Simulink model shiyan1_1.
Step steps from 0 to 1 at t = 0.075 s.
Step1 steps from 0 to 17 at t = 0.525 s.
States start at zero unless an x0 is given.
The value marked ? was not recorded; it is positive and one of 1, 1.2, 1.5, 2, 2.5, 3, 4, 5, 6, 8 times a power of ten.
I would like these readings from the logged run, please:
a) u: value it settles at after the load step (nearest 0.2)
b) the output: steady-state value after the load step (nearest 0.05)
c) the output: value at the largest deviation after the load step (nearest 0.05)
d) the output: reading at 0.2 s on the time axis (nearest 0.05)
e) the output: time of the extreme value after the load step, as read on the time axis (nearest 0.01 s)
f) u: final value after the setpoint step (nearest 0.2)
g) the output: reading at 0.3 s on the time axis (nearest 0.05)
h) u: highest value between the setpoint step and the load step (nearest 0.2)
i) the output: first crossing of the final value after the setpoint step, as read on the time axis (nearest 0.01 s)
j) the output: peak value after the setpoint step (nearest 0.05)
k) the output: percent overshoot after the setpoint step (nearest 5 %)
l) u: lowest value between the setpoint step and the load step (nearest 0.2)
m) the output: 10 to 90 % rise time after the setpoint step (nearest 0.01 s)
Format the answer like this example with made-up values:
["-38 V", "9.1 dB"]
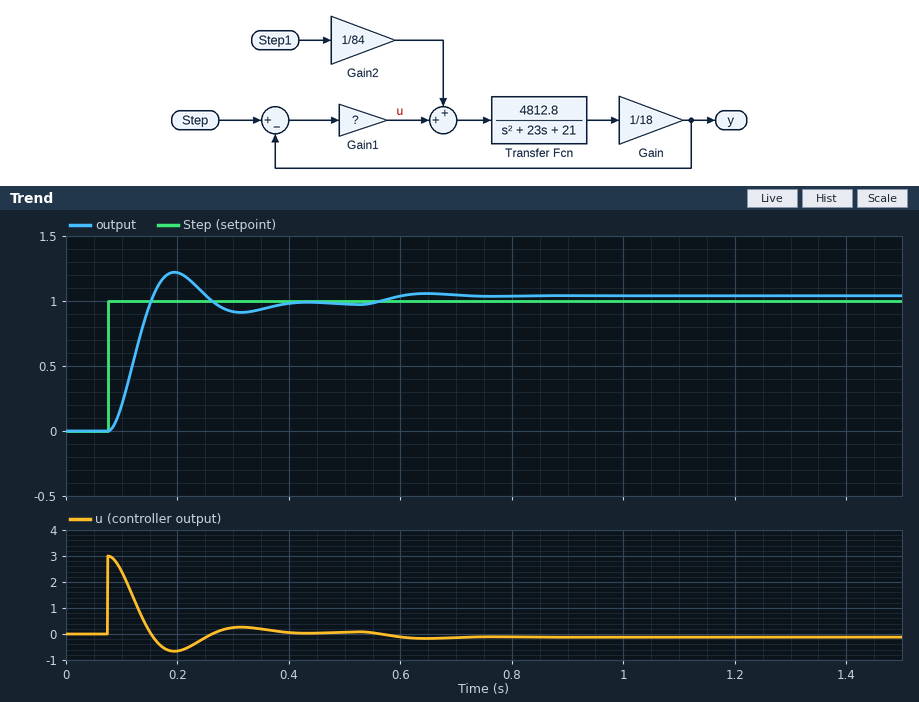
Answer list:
["-0.2", "1.05", "1.05", "1.20", "0.65 s", "0.0", "0.90", "3.0", "0.15 s", "1.20", "25 %", "-0.6", "0.05 s"]
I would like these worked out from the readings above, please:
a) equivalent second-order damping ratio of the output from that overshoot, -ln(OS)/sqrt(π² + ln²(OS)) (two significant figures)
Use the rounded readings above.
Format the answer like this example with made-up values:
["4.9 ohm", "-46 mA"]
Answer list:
["0.40"]
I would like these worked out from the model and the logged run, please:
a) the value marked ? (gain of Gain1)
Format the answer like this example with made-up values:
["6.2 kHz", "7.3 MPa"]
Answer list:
["3"]
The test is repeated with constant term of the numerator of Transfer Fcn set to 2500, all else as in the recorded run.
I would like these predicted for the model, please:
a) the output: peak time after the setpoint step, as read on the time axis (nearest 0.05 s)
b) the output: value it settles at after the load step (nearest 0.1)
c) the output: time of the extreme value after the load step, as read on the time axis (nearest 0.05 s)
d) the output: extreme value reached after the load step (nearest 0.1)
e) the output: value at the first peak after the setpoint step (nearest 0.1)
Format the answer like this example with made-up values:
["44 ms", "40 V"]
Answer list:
["0.25 s", "1.0", "0.70 s", "1.0", "1.1"]
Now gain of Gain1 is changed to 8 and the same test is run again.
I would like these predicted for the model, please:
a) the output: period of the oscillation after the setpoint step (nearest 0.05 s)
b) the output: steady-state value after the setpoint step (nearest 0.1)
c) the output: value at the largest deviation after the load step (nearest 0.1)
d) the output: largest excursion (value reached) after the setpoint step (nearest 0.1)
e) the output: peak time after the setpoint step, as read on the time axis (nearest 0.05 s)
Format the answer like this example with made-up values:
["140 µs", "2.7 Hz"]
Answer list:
["0.15 s", "1.0", "1.0", "1.4", "0.15 s"]
